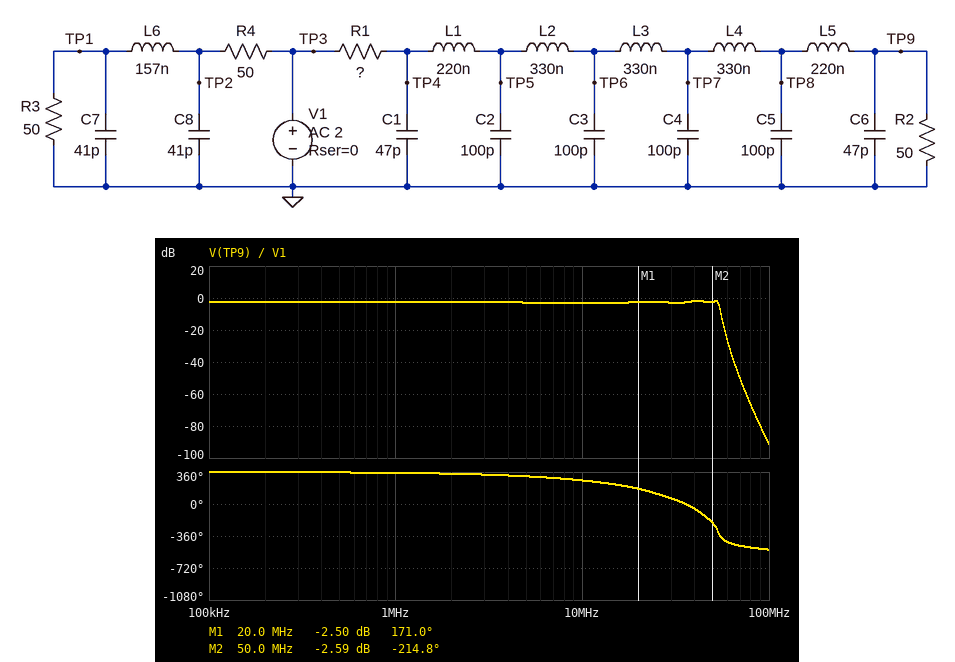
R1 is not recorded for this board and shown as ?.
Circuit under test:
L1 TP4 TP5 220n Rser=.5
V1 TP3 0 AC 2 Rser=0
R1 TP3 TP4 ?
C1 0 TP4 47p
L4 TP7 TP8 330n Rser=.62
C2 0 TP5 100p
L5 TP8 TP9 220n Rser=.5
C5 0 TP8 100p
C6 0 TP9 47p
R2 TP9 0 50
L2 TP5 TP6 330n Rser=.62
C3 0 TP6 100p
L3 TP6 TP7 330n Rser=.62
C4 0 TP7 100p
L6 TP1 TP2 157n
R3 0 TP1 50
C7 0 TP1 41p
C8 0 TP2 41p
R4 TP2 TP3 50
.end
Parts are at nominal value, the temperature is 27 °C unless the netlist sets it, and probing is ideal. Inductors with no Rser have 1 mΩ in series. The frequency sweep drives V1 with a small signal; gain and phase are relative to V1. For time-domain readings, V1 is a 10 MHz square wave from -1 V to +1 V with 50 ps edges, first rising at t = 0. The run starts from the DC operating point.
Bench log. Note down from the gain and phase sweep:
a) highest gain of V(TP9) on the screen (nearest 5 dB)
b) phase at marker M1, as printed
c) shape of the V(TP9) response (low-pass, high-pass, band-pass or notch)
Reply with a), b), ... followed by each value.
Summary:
a) 0 dB
b) 171.0 deg
c) low-pass
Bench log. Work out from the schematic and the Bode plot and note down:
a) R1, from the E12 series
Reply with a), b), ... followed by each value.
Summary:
a) 15 Ω
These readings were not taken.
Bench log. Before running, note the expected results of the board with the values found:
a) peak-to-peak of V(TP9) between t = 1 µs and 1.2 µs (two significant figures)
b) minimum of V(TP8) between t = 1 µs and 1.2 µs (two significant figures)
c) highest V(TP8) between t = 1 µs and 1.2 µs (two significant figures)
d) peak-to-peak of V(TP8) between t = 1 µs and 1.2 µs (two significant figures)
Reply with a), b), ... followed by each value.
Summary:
a) 2.1 V
b) -1.1 V
c) 1.1 V
d) 2.2 V
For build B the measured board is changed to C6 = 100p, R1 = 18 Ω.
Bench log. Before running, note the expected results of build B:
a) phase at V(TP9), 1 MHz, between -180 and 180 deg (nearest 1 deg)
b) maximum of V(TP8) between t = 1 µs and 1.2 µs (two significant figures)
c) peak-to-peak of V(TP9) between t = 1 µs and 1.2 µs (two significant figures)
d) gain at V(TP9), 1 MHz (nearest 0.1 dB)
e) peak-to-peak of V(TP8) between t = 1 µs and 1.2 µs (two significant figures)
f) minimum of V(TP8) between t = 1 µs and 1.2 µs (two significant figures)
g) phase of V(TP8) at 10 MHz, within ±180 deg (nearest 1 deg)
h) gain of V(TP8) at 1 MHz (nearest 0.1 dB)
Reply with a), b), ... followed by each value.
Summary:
a) -10 deg
b) 1.0 V
c) 1.9 V
d) -3.0 dB
e) 2.0 V
f) -1.0 V
g) -86 deg
h) -2.9 dB
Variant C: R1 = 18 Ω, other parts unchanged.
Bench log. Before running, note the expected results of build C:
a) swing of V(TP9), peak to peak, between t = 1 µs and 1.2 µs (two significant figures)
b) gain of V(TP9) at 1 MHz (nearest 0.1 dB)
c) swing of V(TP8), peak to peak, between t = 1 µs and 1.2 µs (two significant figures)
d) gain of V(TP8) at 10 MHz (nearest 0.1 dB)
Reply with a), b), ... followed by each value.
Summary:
a) 2.0 V
b) -3.0 dB
c) 2.1 V
d) -3.4 dB
